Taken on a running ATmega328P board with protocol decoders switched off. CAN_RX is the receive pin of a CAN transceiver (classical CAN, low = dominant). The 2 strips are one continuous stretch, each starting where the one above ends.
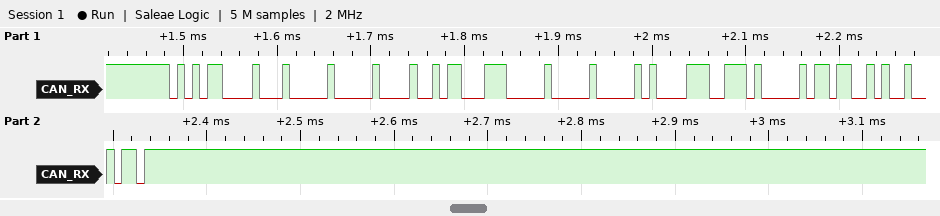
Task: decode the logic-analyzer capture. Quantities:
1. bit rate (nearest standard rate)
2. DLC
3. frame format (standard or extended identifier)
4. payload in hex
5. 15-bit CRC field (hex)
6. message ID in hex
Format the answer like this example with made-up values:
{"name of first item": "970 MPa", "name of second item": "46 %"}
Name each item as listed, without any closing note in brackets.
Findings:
{"bit rate": "125 kbit/s", "DLC": "8", "frame format": "standard", "payload in hex": "00 12 C7 00 00 87 3A 06", "15-bit CRC field": "0x6525", "message ID in hex": "0x561"}
